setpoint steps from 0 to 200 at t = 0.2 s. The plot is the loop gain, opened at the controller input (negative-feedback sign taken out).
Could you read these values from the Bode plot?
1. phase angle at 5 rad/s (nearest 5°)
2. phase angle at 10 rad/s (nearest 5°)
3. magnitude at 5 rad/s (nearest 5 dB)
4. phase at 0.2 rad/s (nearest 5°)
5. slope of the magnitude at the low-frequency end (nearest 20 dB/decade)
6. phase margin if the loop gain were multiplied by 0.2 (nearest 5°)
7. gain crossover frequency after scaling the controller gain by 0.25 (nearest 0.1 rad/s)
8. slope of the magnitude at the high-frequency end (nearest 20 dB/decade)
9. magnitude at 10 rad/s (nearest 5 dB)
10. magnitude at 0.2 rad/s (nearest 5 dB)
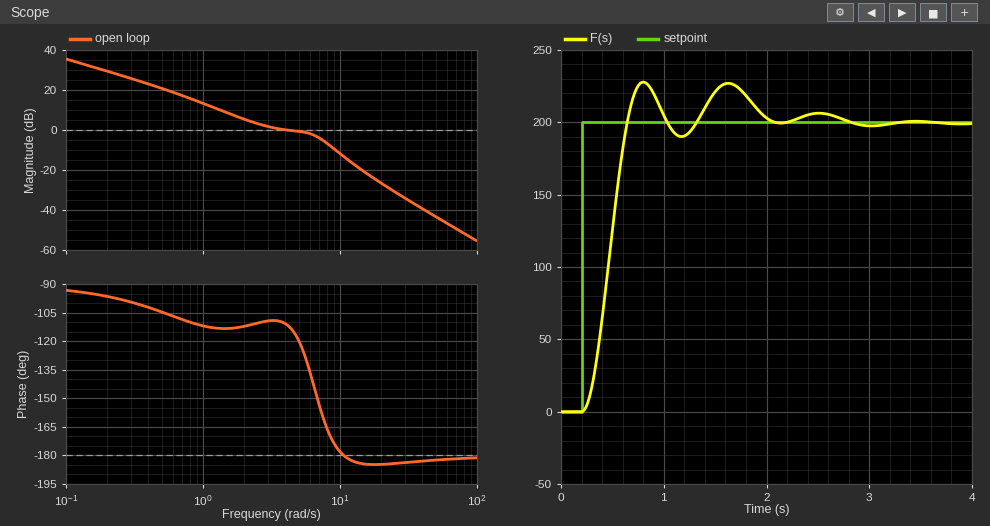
-120°
-180°
0 dB
-95°
-20 dB/decade
70°
1.1 rad/s
-40 dB/decade
-10 dB
30 dB
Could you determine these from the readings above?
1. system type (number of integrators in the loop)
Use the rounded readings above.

1
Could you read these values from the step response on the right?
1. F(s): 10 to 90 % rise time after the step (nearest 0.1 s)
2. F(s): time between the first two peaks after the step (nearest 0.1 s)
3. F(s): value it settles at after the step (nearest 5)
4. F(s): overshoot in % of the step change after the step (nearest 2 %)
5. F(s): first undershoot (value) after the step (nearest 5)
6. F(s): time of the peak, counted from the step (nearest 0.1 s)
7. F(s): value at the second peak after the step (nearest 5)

0.3 s
0.8 s
200
14 %
190
0.6 s
225
